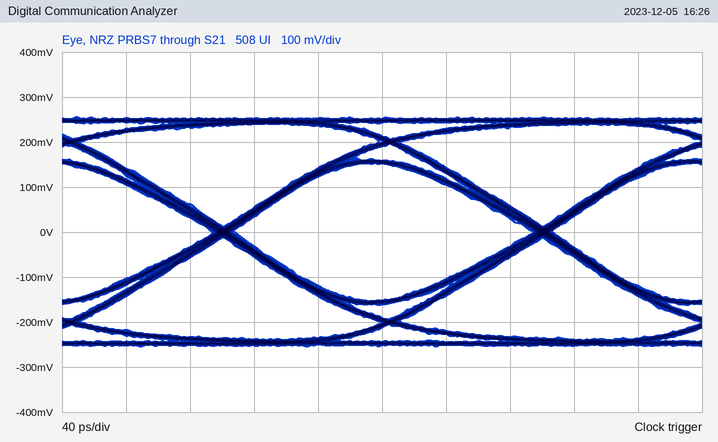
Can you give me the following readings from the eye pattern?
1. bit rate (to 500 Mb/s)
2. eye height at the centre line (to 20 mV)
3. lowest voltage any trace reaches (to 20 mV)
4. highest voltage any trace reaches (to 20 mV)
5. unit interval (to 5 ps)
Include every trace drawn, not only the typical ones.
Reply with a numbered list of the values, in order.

1. 5.0 Gb/s
2. 300 mV
3. -260 mV
4. 260 mV
5. 200 ps
